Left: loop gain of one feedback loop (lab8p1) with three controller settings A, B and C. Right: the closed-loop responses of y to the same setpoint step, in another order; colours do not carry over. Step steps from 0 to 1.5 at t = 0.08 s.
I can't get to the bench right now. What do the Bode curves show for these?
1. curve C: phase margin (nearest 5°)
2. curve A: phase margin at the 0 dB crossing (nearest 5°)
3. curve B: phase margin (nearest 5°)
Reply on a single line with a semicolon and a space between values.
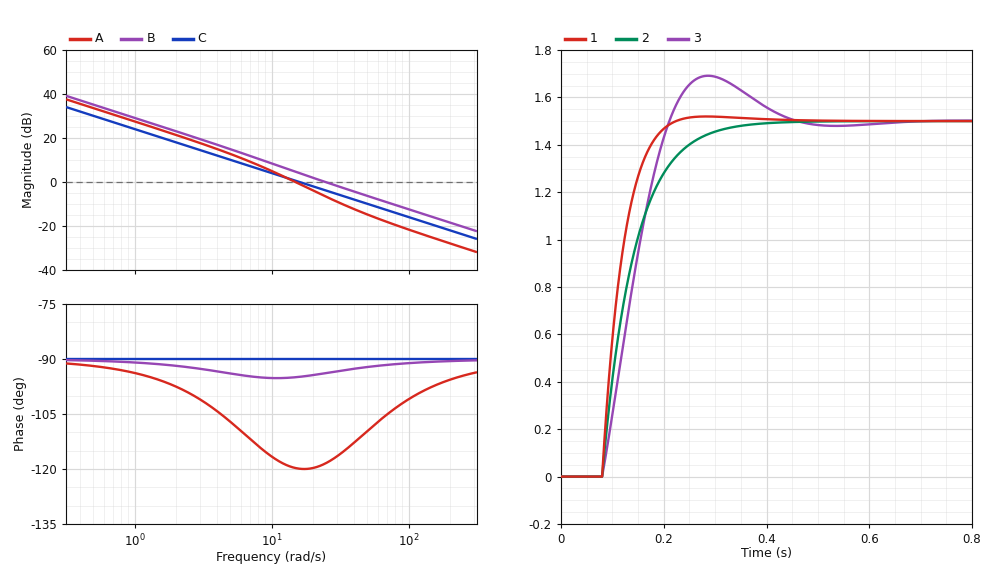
90°; 60°; 85°
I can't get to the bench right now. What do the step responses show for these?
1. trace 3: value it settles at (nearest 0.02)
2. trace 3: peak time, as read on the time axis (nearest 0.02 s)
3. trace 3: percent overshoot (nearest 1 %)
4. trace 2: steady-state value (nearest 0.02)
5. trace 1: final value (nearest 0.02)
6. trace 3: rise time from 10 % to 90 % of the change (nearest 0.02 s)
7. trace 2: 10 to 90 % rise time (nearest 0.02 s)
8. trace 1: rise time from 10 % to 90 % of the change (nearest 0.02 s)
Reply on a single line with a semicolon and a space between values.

1.50; 0.28 s; 13 %; 1.50; 1.50; 0.10 s; 0.14 s; 0.08 s
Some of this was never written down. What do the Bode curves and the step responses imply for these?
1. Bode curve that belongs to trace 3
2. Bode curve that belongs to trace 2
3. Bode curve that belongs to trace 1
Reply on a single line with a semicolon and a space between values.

A; C; B
